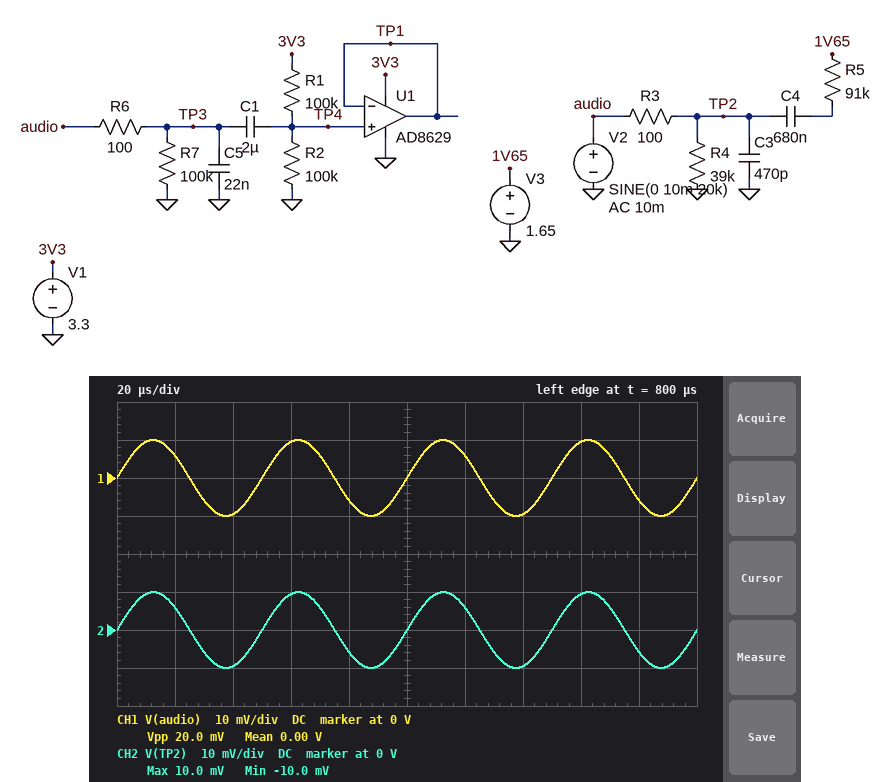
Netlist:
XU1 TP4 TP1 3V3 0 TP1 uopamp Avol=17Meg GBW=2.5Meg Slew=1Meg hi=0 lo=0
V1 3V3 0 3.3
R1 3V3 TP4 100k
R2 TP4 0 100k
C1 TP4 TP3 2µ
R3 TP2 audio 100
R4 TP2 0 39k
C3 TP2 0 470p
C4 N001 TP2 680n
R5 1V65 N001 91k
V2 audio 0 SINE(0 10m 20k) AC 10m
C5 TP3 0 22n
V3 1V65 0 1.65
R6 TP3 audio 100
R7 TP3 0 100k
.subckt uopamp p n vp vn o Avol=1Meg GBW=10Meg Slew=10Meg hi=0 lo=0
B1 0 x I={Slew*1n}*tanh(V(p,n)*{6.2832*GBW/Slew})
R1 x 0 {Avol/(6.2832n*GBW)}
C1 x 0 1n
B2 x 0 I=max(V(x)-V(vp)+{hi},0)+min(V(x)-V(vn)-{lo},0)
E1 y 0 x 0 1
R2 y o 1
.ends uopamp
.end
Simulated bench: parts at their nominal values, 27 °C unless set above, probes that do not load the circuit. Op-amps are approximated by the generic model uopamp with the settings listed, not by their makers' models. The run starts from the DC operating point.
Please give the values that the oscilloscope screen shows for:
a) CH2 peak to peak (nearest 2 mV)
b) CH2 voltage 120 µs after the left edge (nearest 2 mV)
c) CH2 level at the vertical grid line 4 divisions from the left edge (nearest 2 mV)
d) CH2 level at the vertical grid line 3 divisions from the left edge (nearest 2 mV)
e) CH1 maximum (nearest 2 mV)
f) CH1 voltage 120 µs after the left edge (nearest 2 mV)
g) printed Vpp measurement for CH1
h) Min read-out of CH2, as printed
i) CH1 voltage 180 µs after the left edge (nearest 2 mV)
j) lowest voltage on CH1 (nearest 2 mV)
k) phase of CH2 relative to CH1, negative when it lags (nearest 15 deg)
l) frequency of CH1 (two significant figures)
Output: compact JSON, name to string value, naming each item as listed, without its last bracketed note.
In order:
{"CH2 peak to peak": "20 mV", "CH2 voltage 120 µs after the left edge": "6 mV", "CH2 level at the vertical grid line 4 divisions from the left edge": "-6 mV", "CH2 level at the vertical grid line 3 divisions from the left edge": "10 mV", "CH1 maximum": "10 mV", "CH1 voltage 120 µs after the left edge": "6 mV", "printed Vpp measurement for CH1": "20.0 mV", "Min read-out of CH2, as printed": "-10.0 mV", "CH1 voltage 180 µs after the left edge": "-6 mV", "lowest voltage on CH1": "-10 mV", "phase of CH2 relative to CH1, negative when it lags": "0 deg", "frequency of CH1": "20 kHz"}
